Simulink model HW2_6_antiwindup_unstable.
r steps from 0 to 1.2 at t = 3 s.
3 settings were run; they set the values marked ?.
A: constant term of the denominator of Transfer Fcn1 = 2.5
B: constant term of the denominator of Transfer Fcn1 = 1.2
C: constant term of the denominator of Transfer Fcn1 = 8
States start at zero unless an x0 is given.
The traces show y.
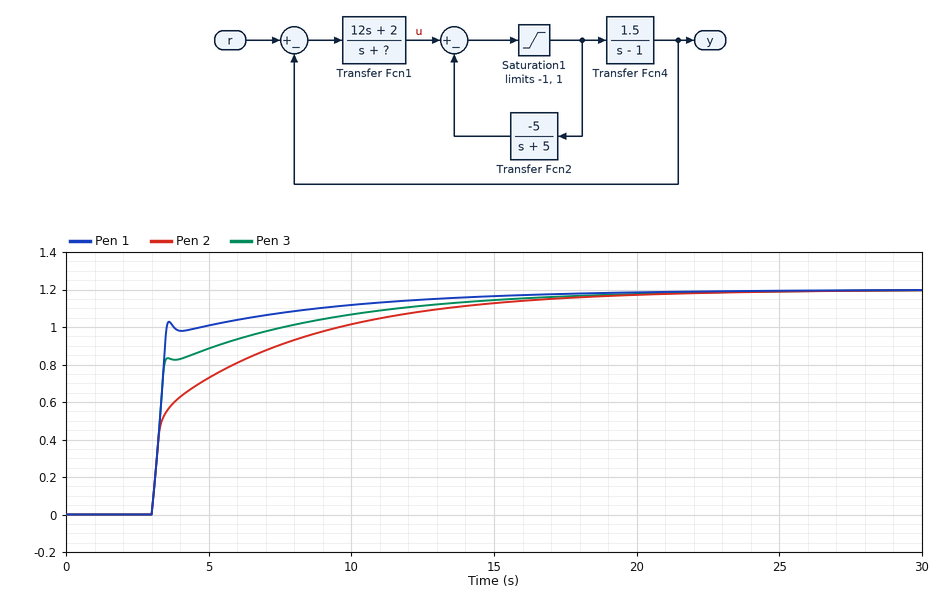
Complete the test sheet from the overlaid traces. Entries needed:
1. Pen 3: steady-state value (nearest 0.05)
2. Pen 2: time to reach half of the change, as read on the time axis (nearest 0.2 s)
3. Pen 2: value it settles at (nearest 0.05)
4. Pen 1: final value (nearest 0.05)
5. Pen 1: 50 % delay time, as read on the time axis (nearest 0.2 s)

1.20
3.8 s
1.20
1.20
3.4 s
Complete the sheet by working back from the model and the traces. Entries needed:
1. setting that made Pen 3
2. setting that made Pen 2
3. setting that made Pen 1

A
C
B
